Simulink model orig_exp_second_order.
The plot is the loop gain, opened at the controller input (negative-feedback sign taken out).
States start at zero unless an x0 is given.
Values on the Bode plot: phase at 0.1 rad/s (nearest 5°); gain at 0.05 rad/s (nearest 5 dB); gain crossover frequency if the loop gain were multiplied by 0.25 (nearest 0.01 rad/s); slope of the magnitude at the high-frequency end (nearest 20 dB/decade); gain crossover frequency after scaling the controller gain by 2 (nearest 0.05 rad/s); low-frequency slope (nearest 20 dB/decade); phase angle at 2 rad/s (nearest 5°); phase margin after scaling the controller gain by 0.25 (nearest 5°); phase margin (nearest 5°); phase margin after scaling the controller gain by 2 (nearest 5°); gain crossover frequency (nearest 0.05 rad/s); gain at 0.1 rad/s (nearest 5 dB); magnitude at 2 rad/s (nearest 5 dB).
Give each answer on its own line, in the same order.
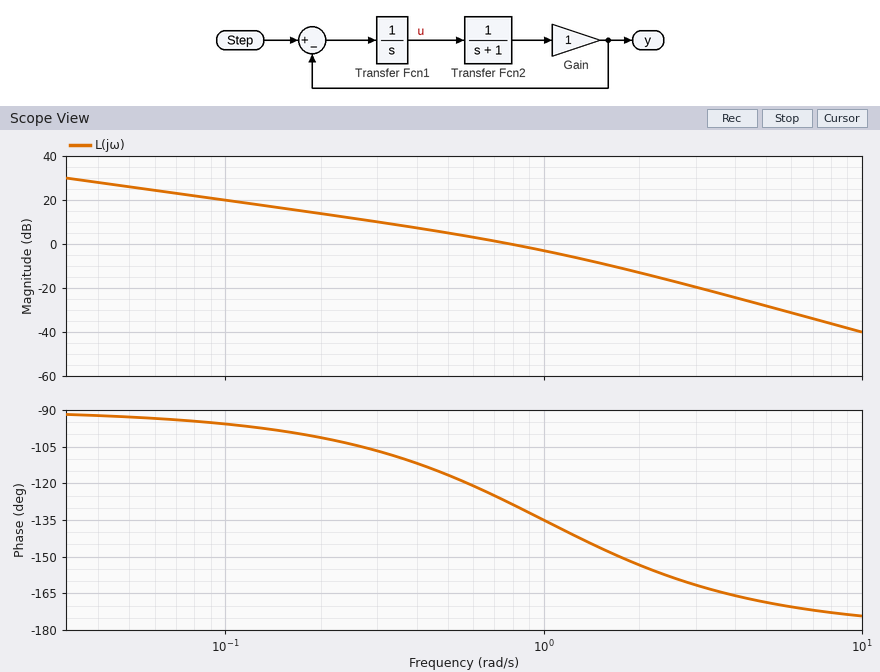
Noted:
-95°
25 dB
0.24 rad/s
-40 dB/decade
1.25 rad/s
-20 dB/decade
-155°
75°
50°
40°
0.80 rad/s
20 dB
-15 dB
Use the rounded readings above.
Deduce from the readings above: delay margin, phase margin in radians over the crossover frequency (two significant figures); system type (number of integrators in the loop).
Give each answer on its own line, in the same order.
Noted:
1.1 s
1
